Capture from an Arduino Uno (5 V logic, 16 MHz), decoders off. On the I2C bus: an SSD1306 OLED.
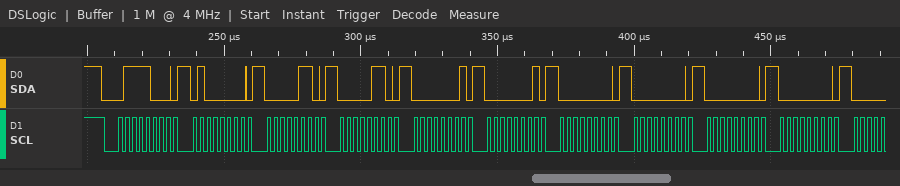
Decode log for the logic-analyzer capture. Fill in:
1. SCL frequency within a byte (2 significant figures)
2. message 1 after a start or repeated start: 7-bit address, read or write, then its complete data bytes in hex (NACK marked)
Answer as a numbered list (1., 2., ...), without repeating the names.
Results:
1. 400 kHz
2. 0x3C write: 40 06 06 01 01 00 00 00 00
